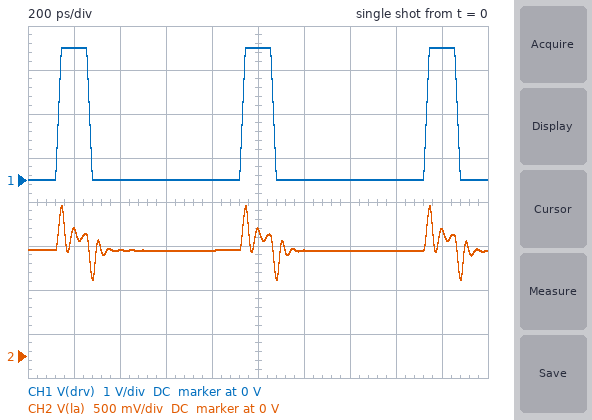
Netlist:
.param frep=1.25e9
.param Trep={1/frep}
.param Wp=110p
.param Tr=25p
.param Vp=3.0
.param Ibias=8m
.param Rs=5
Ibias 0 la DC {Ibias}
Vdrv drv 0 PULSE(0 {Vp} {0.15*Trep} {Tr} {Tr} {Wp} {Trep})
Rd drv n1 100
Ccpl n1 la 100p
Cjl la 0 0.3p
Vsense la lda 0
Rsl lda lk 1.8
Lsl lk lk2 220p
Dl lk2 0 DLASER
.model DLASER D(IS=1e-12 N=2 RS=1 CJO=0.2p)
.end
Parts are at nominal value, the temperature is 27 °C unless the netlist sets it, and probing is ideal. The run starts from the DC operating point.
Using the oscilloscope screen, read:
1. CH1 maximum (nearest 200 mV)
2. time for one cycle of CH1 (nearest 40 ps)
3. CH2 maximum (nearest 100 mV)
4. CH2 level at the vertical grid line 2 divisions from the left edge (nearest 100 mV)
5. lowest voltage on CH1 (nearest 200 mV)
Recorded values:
3.0 V
800 ps
1.7 V
1.2 V
0 V
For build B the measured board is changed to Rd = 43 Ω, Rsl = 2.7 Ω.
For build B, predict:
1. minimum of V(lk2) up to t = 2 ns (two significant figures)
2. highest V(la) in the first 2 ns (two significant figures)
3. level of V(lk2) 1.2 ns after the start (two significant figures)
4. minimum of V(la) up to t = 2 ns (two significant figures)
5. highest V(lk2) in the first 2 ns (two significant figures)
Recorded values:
1.0 V
2.2 V
1.2 V
610 mV
1.4 V
